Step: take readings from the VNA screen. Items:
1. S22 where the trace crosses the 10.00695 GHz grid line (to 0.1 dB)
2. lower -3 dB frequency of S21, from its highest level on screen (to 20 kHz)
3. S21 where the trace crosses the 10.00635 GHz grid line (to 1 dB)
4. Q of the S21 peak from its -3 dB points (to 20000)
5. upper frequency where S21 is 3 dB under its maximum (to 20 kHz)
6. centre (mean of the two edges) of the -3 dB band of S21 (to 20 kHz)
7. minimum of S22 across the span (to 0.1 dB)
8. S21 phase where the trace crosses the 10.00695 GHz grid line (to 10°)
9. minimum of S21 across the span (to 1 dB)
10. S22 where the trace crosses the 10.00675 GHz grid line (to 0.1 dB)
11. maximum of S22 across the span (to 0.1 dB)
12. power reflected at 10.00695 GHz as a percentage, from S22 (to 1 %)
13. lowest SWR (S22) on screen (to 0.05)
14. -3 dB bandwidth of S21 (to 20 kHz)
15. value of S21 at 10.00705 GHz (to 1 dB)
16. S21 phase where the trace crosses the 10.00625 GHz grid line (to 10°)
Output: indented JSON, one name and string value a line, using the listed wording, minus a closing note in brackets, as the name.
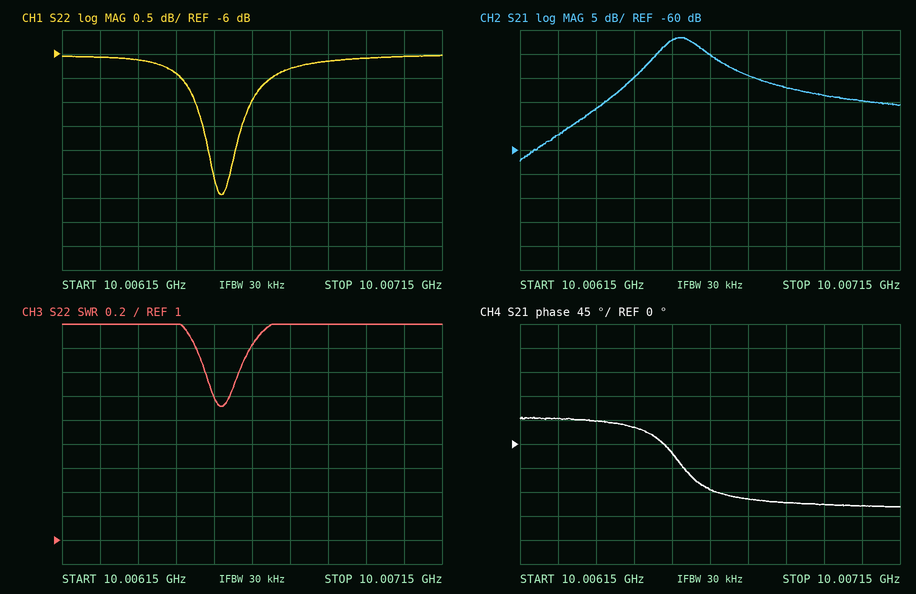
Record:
{
  "S22 where the trace crosses the 10.00695 GHz grid line": "-6.1 dB",
  "lower -3 dB frequency of S21, from its highest level on screen": "10.00652 GHz",
  "S21 where the trace crosses the 10.00635 GHz grid line": "-51 dB",
  "Q of the S21 peak from its -3 dB points": "80000",
  "upper frequency where S21 is 3 dB under its maximum": "10.00664 GHz",
  "centre (mean of the two edges) of the -3 dB band of S21": "10.00658 GHz",
  "minimum of S22 across the span": "-8.9 dB",
  "S21 phase where the trace crosses the 10.00695 GHz grid line": "-110°",
  "minimum of S21 across the span": "-62 dB",
  "S22 where the trace crosses the 10.00675 GHz grid line": "-6.3 dB",
  "maximum of S22 across the span": "-6.0 dB",
  "power reflected at 10.00695 GHz as a percentage, from S22": "25 %",
  "lowest SWR (S22) on screen": "2.10",
  "-3 dB bandwidth of S21": "120 kHz",
  "value of S21 at 10.00705 GHz": "-50 dB",
  "S21 phase where the trace crosses the 10.00625 GHz grid line": "50°"
}
